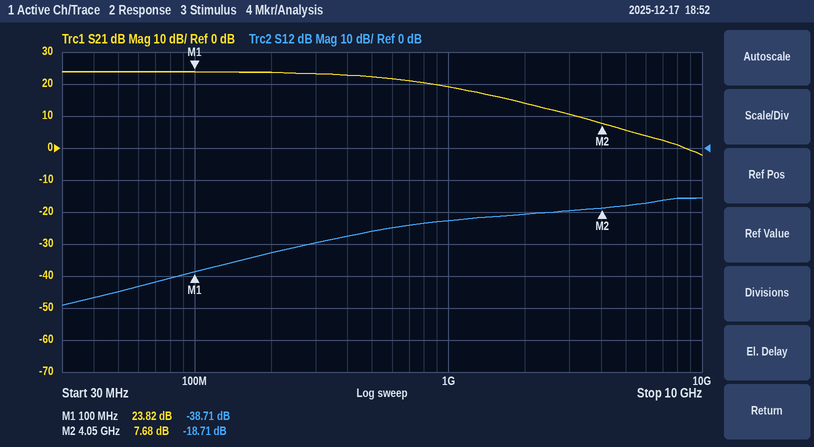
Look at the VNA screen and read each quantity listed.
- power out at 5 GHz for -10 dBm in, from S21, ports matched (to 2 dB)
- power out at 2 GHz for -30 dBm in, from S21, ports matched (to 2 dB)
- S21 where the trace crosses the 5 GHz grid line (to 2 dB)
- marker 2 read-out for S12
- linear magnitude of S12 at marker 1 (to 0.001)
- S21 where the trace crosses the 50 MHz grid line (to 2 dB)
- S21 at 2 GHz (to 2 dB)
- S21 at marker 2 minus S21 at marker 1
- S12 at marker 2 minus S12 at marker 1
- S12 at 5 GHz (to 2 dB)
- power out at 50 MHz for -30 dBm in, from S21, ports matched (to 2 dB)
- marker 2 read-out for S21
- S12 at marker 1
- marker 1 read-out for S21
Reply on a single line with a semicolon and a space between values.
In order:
-4 dBm; -16 dBm; 6 dB; -18.71 dB; 0.012; 24 dB; 14 dB; -16.14 dB; 20.00 dB; -18 dB; -6 dBm; 7.68 dB; -38.71 dB; 23.82 dB
